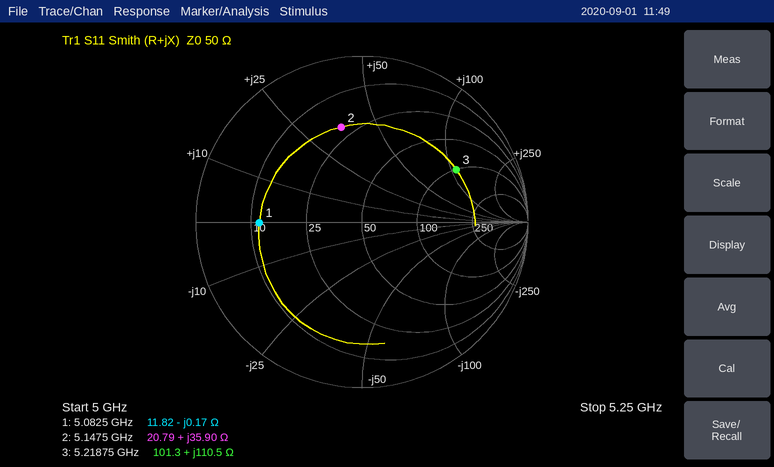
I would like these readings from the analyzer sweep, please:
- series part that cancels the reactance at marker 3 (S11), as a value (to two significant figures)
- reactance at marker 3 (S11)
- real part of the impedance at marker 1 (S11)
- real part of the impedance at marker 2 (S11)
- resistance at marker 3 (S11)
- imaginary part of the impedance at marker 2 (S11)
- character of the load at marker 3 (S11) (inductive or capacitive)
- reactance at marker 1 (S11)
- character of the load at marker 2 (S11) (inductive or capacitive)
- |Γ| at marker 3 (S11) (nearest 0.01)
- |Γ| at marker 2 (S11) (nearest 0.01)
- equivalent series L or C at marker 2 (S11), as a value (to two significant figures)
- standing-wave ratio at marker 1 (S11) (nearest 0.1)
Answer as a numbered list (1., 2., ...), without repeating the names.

1. 280 fF
2. +110.5 Ω
3. 11.82 Ω
4. 20.79 Ω
5. 101.3 Ω
6. +35.90 Ω
7. inductive
8. -0.17 Ω
9. inductive
10. 0.65
11. 0.58
12. 1.1 nH
13. 4.2
